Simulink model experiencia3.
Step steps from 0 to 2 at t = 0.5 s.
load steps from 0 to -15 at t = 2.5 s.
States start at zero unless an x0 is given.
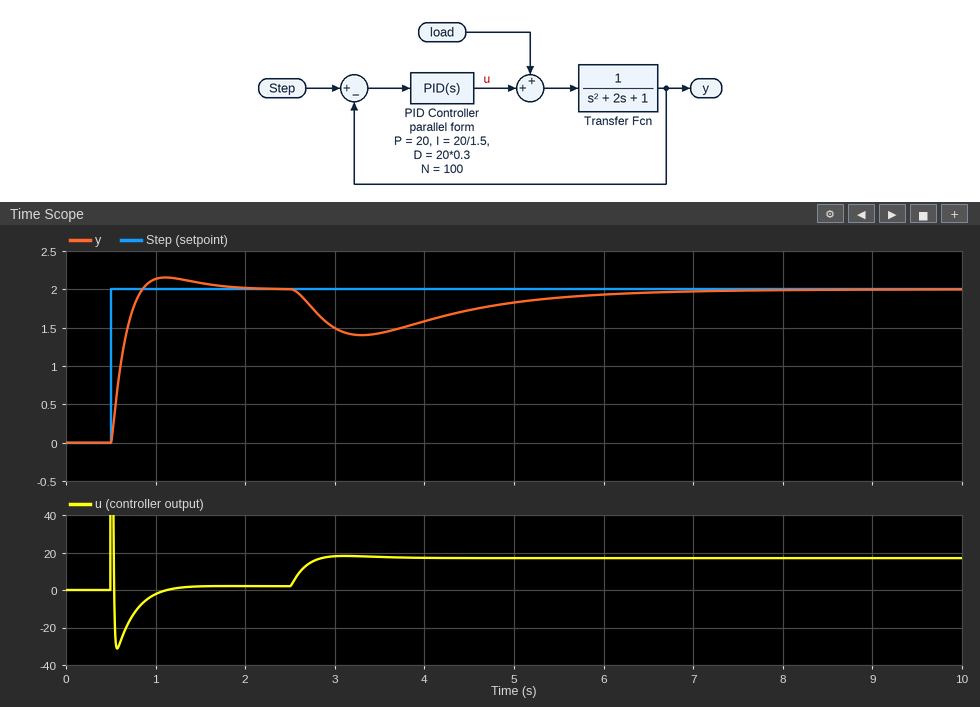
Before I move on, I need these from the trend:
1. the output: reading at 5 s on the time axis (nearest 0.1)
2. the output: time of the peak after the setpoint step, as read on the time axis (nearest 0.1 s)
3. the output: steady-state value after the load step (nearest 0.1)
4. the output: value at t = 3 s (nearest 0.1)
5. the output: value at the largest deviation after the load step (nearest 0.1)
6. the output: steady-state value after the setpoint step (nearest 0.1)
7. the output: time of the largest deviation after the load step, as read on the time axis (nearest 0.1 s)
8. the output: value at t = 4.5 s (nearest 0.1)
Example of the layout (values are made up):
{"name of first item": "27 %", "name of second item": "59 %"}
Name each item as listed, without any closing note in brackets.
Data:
{"the output: reading at 5 s on the time axis": "1.8", "the output: time of the peak after the setpoint step, as read on the time axis": "1.1 s", "the output: steady-state value after the load step": "2.0", "the output: value at t = 3 s": "1.5", "the output: value at the largest deviation after the load step": "1.4", "the output: steady-state value after the setpoint step": "2.0", "the output: time of the largest deviation after the load step, as read on the time axis": "3.3 s", "the output: value at t = 4.5 s": "1.7"}
